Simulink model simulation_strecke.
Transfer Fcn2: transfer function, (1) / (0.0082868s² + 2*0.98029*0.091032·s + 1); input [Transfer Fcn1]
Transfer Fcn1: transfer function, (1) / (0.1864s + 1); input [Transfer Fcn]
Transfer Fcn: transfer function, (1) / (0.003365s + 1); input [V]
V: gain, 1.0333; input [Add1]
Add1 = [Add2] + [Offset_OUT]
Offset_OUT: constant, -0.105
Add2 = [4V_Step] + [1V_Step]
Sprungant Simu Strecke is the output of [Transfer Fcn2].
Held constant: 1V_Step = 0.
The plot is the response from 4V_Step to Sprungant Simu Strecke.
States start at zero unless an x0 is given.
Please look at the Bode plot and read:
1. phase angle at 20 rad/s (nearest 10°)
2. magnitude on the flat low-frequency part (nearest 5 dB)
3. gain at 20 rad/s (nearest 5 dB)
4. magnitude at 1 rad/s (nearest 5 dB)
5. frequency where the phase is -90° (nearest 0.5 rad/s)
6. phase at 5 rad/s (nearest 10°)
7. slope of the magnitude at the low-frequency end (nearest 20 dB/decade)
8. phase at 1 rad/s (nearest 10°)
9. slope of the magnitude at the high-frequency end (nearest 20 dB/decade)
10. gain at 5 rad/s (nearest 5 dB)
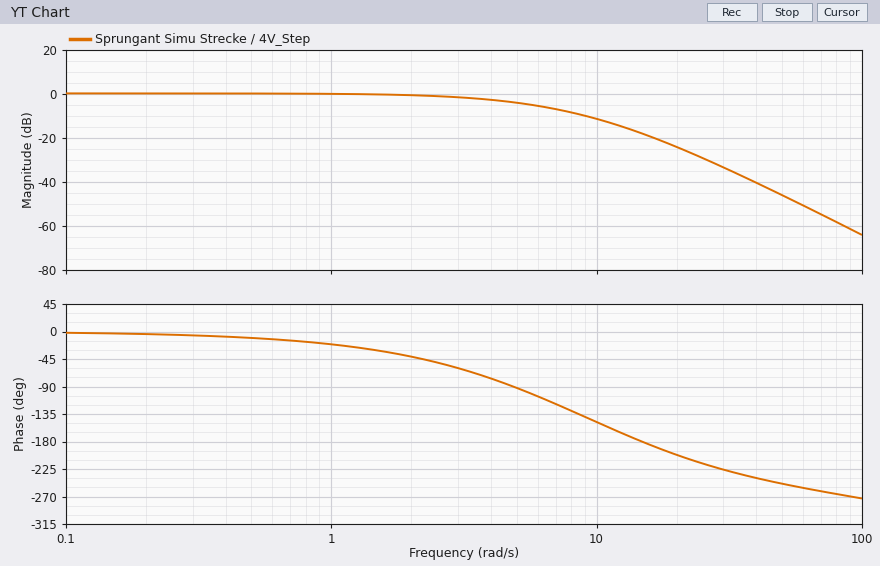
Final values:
-200°
0 dB
-25 dB
0 dB
5.0 rad/s
-90°
0 dB/decade
-20°
-60 dB/decade
-5 dB
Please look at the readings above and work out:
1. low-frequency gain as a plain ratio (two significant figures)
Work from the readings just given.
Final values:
1.0
